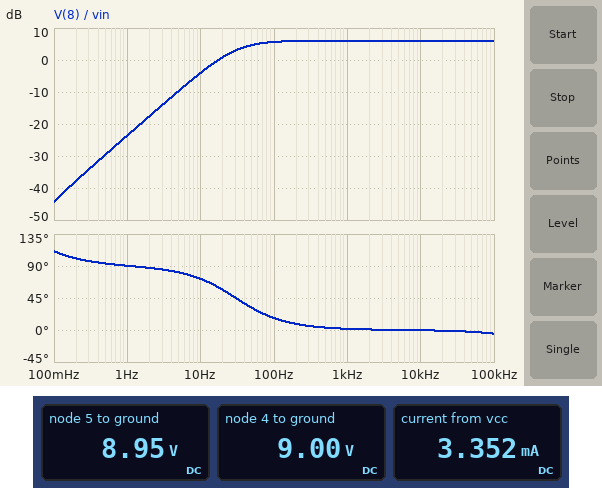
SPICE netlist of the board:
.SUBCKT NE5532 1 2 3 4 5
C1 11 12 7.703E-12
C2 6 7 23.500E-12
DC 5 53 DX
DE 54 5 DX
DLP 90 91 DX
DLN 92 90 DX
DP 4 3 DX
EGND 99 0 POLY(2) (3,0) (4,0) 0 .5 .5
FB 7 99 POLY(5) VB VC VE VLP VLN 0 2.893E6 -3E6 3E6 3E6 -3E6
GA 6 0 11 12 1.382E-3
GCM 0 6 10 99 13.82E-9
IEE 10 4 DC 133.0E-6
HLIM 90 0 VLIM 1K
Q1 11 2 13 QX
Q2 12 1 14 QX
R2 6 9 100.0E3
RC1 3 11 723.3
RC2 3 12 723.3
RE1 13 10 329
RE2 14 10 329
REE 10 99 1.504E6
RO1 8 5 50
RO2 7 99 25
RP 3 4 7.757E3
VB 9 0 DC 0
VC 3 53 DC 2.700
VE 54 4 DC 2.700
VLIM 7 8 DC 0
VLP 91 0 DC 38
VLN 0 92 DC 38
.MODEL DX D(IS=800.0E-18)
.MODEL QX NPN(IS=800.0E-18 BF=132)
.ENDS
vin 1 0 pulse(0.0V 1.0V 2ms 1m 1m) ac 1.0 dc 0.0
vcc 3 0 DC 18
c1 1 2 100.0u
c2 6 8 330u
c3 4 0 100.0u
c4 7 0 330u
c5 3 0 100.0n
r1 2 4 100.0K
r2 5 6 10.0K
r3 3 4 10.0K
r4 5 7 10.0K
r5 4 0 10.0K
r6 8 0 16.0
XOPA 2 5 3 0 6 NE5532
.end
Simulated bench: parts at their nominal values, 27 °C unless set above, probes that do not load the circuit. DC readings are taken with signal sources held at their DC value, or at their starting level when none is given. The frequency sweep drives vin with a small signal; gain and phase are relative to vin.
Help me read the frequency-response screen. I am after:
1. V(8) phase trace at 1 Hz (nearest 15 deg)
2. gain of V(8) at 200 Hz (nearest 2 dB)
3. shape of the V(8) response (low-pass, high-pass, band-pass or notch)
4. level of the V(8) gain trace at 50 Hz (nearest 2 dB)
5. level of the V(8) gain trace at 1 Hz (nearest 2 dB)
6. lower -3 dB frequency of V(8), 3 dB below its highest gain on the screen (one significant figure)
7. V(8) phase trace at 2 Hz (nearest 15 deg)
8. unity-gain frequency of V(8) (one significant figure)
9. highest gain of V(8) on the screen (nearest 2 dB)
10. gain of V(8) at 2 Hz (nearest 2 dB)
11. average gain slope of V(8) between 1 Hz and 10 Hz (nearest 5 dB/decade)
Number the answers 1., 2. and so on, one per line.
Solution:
1. 90 deg
2. 6 dB
3. high-pass
4. 4 dB
5. -24 dB
6. 30 Hz
7. 90 deg
8. 20 Hz
9. 6 dB
10. -18 dB
11. 20 dB/decade
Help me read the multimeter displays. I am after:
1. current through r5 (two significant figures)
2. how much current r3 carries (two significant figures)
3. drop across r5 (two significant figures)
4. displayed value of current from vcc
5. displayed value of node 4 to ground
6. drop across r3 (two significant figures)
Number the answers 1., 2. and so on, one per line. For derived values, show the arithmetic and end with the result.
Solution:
1. (9 V) / 10 kΩ = 900 µA
2. (18 V - 9 V) / 10 kΩ = 900 µA
3. 9 V = 9.0 V
4. 3.352 mA
5. 9.00 V
6. 18 V - 9 V = 9.0 V
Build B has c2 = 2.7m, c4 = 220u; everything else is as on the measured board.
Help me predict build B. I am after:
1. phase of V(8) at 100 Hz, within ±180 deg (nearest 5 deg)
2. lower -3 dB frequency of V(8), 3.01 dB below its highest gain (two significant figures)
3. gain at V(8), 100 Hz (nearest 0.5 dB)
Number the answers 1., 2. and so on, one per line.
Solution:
1. 0 deg
2. 3.7 Hz
3. 6.0 dB
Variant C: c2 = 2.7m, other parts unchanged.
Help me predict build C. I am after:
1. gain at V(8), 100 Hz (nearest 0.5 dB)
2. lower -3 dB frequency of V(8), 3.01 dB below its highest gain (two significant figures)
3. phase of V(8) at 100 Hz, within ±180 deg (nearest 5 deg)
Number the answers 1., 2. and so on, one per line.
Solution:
1. 6.0 dB
2. 3.7 Hz
3. 0 deg
